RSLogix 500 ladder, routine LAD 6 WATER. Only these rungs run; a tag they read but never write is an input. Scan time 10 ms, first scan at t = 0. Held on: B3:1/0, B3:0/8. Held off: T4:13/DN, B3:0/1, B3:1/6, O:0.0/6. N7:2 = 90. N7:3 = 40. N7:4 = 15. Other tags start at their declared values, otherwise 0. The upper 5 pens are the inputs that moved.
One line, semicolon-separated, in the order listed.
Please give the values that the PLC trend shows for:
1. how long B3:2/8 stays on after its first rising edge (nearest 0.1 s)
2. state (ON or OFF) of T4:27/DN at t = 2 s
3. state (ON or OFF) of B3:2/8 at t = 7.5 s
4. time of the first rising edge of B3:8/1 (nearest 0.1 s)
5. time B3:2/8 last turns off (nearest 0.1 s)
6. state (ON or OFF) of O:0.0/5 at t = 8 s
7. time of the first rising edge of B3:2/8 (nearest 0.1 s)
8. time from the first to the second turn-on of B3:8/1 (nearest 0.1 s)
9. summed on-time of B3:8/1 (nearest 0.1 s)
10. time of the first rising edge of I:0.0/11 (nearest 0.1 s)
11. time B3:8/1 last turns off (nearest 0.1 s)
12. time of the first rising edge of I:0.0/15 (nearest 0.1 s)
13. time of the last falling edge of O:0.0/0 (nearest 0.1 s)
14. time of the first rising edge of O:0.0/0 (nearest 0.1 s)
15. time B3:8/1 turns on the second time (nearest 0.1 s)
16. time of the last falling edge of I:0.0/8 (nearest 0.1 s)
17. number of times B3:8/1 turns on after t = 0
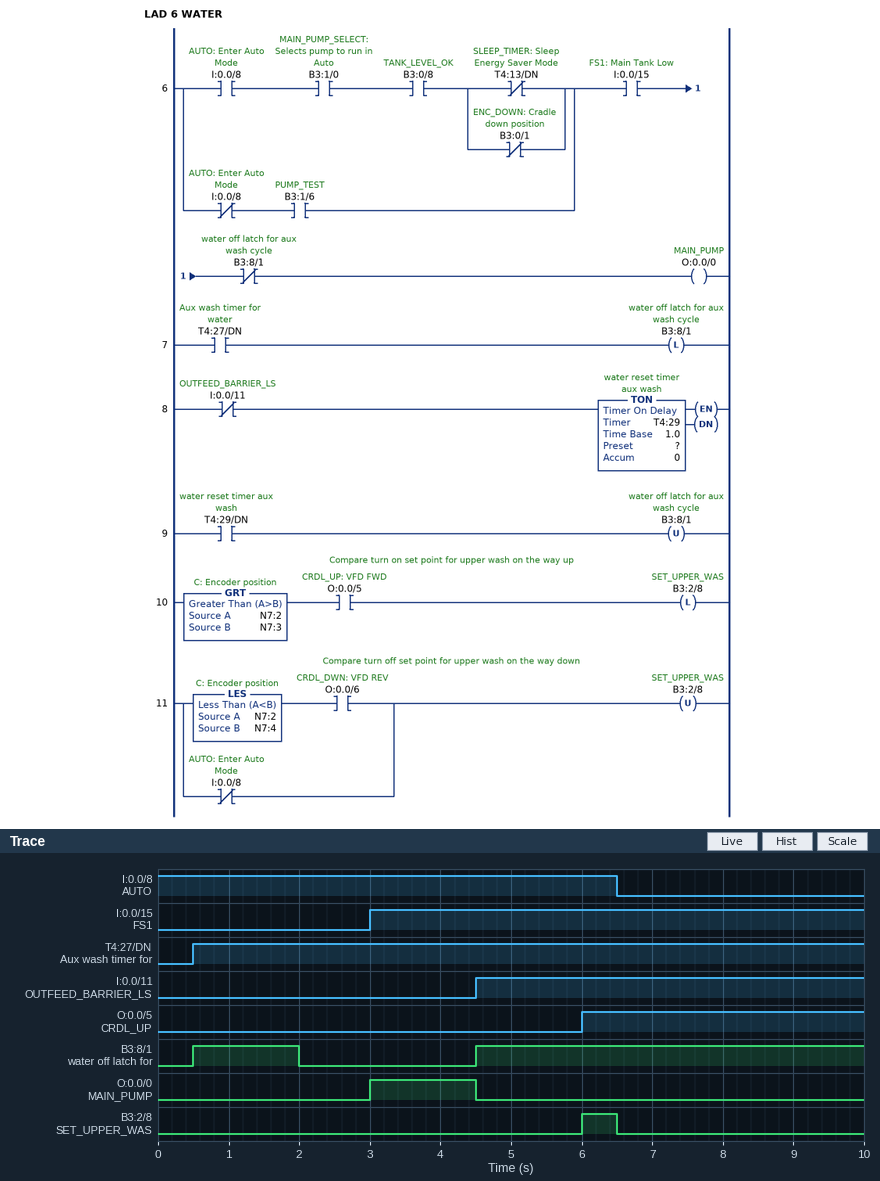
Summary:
0.5 s; ON; OFF; 0.5 s; 6.5 s; ON; 6.0 s; 4.0 s; 7.0 s; 4.5 s; 2.0 s; 3.0 s; 4.5 s; 3.0 s; 4.5 s; 6.5 s; 2
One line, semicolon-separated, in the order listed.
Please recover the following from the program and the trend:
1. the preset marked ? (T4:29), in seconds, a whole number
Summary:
2 s
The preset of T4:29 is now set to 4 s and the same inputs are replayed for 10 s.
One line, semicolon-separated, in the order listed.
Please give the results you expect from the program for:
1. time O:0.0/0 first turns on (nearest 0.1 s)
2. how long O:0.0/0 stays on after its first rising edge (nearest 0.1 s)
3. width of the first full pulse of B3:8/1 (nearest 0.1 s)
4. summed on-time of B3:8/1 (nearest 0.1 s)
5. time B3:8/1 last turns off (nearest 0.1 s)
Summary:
4.0 s; 0.5 s; 3.5 s; 9.0 s; 4.0 s
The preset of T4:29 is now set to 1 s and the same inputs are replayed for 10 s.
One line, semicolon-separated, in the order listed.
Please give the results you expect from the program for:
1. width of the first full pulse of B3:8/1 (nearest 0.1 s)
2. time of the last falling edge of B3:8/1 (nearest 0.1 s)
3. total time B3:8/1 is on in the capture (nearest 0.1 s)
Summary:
0.5 s; 1.0 s; 6.0 s
